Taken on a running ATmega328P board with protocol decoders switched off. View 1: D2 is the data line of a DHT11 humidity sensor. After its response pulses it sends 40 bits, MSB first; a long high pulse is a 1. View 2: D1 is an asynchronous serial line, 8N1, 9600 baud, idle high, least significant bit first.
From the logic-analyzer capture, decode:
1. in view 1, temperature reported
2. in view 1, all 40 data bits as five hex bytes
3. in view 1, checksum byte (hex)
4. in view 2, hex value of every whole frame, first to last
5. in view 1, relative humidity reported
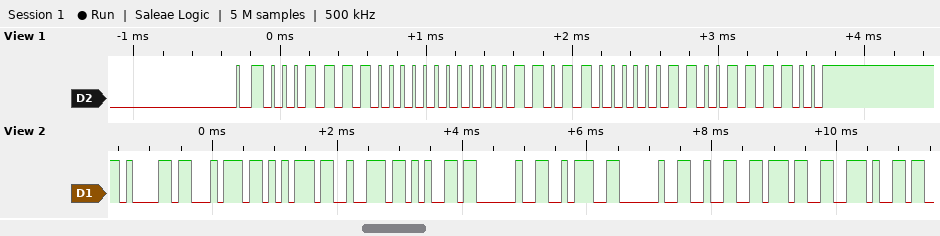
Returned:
27.3 °C
1E 00 1B 03 3C
0x3C
61 74 75 72 65 20 3A 20 32 37 2E
30 %
